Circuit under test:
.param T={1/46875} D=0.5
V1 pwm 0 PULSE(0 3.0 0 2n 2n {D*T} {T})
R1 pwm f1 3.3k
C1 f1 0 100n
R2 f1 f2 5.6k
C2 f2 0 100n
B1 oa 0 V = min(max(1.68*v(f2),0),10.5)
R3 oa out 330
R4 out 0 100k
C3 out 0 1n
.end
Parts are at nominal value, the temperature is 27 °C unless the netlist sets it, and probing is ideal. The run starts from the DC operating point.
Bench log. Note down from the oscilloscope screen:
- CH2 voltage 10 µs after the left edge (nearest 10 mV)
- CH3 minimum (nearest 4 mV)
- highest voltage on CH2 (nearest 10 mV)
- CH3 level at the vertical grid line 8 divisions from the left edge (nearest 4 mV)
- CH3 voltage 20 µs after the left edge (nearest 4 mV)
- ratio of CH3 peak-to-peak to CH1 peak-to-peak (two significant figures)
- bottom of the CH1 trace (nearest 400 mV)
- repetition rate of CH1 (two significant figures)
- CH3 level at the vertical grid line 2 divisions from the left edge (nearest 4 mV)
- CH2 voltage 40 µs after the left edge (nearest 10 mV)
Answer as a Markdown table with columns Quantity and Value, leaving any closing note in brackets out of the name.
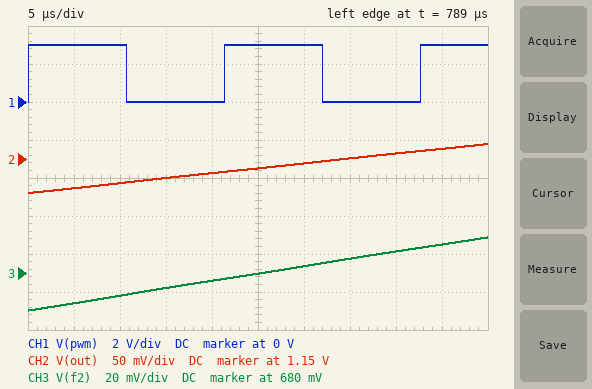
| Quantity | Value |
|---|---|
| CH2 voltage 10 µs after the left edge | 1.12 V |
| CH3 minimum | 660 mV |
| highest voltage on CH2 | 1.17 V |
| CH3 level at the vertical grid line 8 divisions from the left edge | 692 mV |
| CH3 voltage 20 µs after the left edge | 676 mV |
| ratio of CH3 peak-to-peak to CH1 peak-to-peak | 0.013 |
| bottom of the CH1 trace | 0 V |
| repetition rate of CH1 | 47 kHz |
| CH3 level at the vertical grid line 2 divisions from the left edge | 668 mV |
| CH2 voltage 40 µs after the left edge | 1.16 V |
